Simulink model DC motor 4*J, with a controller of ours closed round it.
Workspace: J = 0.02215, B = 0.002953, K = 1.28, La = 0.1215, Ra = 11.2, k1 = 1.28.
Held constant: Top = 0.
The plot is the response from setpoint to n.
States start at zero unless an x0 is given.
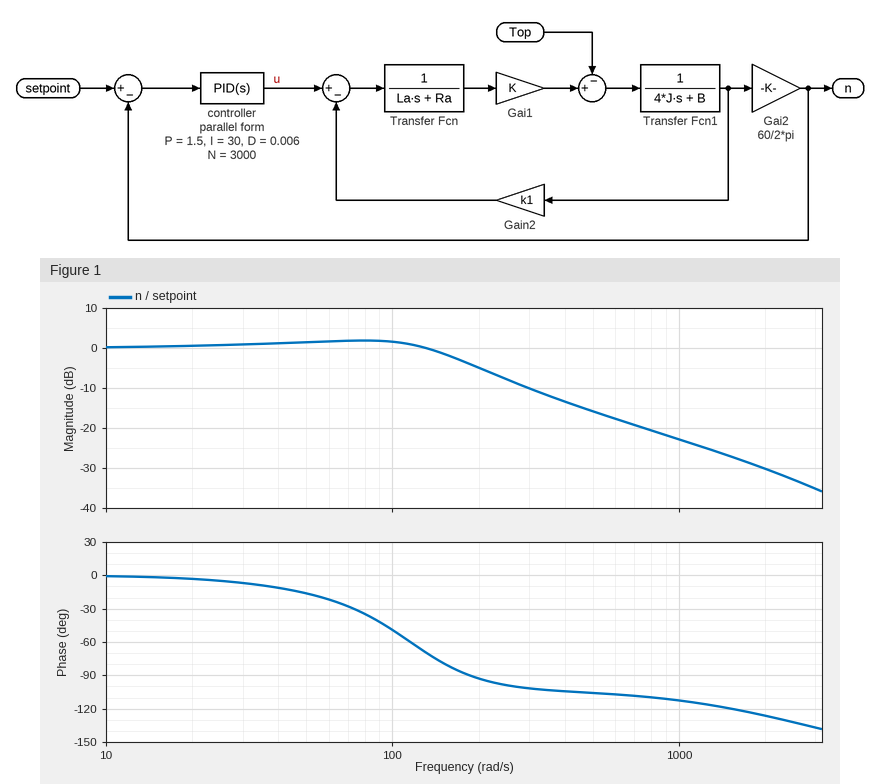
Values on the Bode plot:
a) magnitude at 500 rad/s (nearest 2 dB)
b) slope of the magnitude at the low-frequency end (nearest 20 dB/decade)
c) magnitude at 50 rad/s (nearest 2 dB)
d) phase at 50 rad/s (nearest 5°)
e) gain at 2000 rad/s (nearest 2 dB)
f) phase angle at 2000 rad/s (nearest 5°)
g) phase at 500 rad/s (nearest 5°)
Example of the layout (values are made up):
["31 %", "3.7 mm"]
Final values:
["-16 dB", "0 dB/decade", "2 dB", "-15°", "-30 dB", "-125°", "-105°"]
